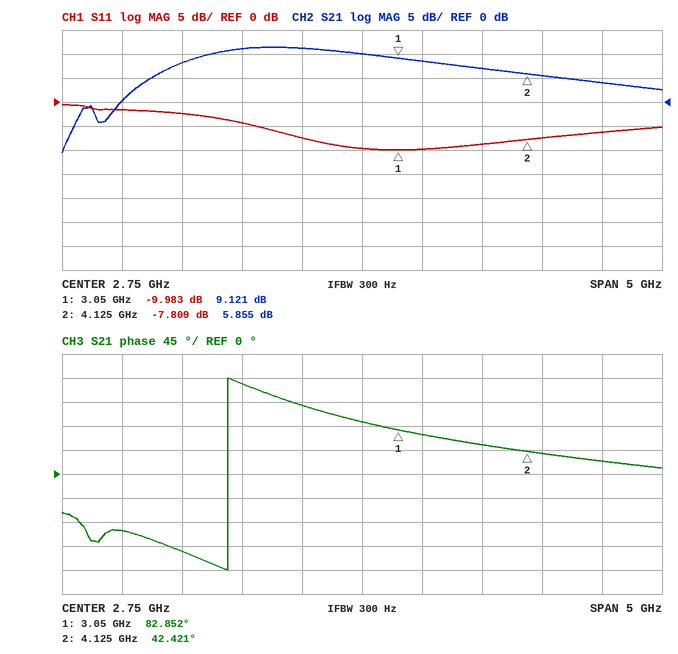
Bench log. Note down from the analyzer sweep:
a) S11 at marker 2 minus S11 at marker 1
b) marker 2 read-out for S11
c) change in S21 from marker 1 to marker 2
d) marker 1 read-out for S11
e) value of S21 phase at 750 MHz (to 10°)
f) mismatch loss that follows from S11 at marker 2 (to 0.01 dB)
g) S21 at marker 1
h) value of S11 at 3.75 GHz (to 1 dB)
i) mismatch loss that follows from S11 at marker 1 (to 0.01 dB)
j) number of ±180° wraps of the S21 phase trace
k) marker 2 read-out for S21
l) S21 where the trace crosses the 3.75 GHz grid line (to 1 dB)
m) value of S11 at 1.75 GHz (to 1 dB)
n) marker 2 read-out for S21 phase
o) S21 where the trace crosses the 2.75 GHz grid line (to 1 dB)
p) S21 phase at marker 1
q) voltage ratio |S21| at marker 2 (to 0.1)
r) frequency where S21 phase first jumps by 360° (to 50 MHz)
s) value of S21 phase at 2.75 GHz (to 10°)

2.174 dB
-7.809 dB
-3.266 dB
-9.983 dB
-110°
0.79 dB
9.121 dB
-9 dB
0.46 dB
1
5.855 dB
7 dB
-4 dB
42.421°
10 dB
82.852°
2.0
1.65 GHz
100°
